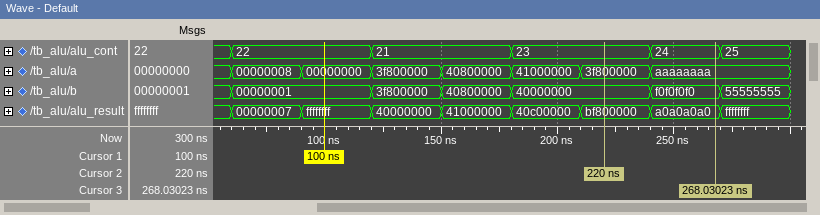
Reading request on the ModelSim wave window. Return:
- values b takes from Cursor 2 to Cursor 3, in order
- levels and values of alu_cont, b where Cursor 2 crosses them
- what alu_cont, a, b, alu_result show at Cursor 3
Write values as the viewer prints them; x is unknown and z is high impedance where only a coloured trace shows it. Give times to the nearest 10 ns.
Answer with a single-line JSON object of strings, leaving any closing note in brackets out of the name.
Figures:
{"values b takes from Cursor 2 to Cursor 3, in order": "40000000, f0f0f0f0", "levels and values of alu_cont, b where Cursor 2 crosses them": "alu_cont=23, b=40000000", "what alu_cont, a, b, alu_result show at Cursor 3": "alu_cont=24, a=aaaaaaaa, b=f0f0f0f0, alu_result=a0a0a0a0"}
